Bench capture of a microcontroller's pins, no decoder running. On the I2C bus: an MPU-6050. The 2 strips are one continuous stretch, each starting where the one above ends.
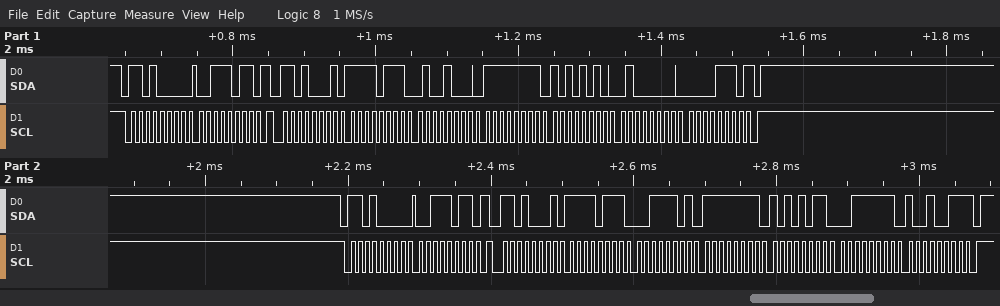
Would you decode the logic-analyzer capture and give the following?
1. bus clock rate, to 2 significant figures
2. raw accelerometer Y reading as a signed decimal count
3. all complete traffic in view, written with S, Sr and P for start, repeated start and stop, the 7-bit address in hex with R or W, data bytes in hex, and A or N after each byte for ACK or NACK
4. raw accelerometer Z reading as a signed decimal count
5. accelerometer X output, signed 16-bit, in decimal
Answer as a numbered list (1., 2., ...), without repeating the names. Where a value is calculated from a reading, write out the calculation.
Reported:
1. 100 kHz
2. 0xFFAA = -86
3. S 68W A 3B A Sr 68R A F7 A 48 A FF A AA A 40 A 0E N P S 68W A 3B A Sr 68R A F7 A 3D A FF A AB A 3F A 93 N P
4. 0x400E = 16398
5. 0xF748 = -2232
